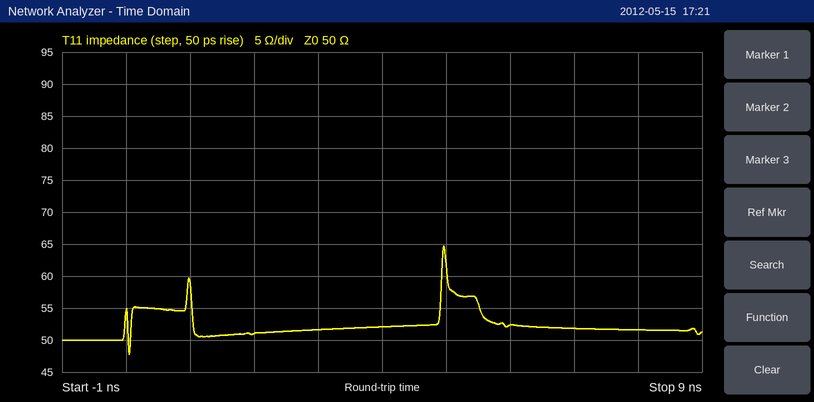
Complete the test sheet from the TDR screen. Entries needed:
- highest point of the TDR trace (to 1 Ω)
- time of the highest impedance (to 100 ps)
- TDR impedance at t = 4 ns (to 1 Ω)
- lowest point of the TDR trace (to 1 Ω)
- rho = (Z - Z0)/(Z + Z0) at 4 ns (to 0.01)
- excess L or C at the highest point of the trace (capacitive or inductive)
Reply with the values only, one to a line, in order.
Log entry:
65 Ω
5.0 ns
52 Ω
48 Ω
+0.02
inductive
